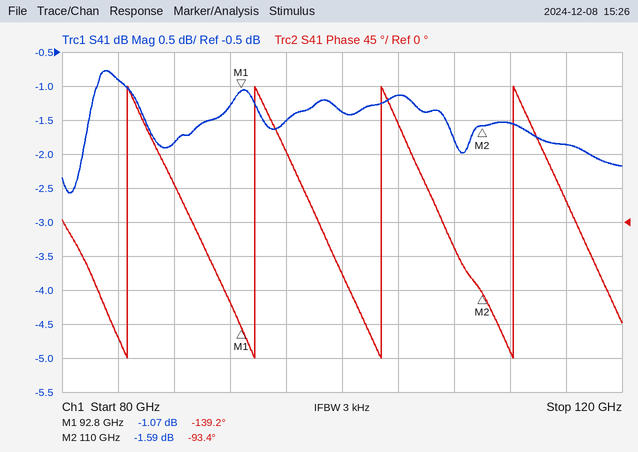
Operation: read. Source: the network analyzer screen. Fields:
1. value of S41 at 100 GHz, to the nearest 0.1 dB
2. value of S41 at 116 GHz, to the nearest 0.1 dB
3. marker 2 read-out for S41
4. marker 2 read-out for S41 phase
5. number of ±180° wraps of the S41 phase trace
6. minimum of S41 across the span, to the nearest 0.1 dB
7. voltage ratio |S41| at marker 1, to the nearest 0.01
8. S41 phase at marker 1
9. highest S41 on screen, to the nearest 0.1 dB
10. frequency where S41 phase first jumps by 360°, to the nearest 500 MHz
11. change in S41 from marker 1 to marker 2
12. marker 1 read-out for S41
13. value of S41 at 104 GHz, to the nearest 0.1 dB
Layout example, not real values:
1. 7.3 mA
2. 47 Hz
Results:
1. -1.4 dB
2. -1.9 dB
3. -1.59 dB
4. -93.4°
5. 4
6. -2.6 dB
7. 0.88
8. -139.2°
9. -0.8 dB
10. 84.5 GHz
11. -0.52 dB
12. -1.07 dB
13. -1.1 dB
